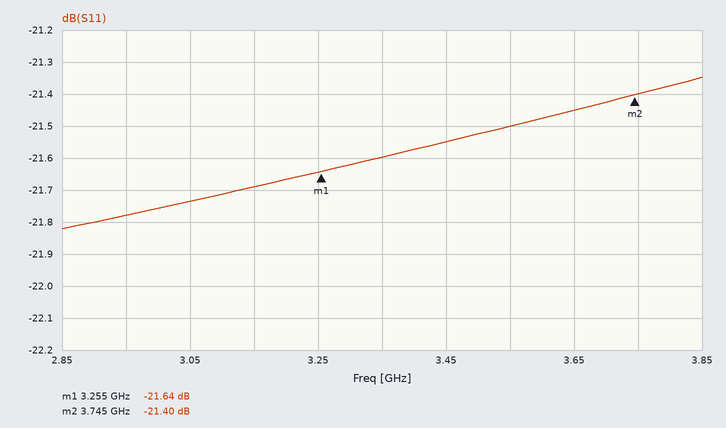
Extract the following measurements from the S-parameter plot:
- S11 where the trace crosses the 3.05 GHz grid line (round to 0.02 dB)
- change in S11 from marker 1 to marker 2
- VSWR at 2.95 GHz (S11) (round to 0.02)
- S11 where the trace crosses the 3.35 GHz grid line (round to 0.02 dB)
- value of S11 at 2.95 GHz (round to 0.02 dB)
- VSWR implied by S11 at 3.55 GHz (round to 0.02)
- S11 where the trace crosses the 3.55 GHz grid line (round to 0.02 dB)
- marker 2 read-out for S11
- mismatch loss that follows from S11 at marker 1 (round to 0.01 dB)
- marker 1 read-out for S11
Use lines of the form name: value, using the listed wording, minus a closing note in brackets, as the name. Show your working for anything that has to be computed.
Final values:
S11 where the trace crosses the 3.05 GHz grid line: -21.74 dB
change in S11 from marker 1 to marker 2: -21.4 − (-21.64) = 0.24 dB
VSWR at 2.95 GHz (S11): |Γ| = 10^(-21.78/20) = 0.0815; VSWR = (1 + 0.0815)/(1 − 0.0815) ≈ 1.18
S11 where the trace crosses the 3.35 GHz grid line: -21.60 dB
value of S11 at 2.95 GHz: -21.78 dB
VSWR implied by S11 at 3.55 GHz: |Γ| = 10^(-21.5/20) = 0.0841; VSWR = (1 + 0.0841)/(1 − 0.0841) ≈ 1.18
S11 where the trace crosses the 3.55 GHz grid line: -21.50 dB
marker 2 read-out for S11: -21.40 dB
mismatch loss that follows from S11 at marker 1: −10 log10(1 − 10^(-21.64/10)) ≈ 0.03 dB
marker 1 read-out for S11: -21.64 dB
